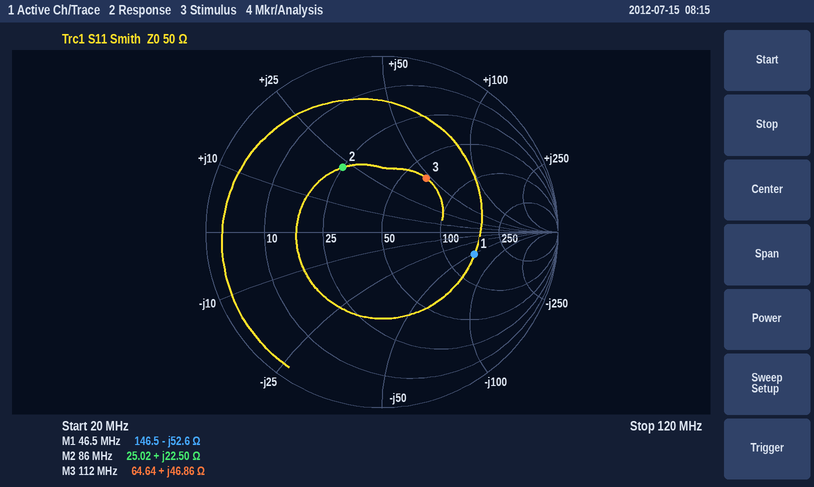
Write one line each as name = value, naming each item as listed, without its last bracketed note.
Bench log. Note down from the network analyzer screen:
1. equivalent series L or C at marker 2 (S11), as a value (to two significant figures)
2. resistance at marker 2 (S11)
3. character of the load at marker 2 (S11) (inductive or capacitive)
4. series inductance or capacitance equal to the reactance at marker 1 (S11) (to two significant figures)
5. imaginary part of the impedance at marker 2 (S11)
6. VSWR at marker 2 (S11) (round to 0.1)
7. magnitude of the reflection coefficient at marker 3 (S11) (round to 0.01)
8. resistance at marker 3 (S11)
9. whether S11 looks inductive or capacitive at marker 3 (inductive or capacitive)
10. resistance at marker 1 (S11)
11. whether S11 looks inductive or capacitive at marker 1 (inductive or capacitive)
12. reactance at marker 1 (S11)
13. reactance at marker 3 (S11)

equivalent series L or C at marker 2 (S11), as a value = 42 nH
resistance at marker 2 = 25.02 Ω
character of the load at marker 2 (S11) = inductive
series inductance or capacitance equal to the reactance at marker 1 (S11) = 65 pF
imaginary part of the impedance at marker 2 = +22.50 Ω
VSWR at marker 2 (S11) = 2.5
magnitude of the reflection coefficient at marker 3 (S11) = 0.40
resistance at marker 3 = 64.64 Ω
whether S11 looks inductive or capacitive at marker 3 = inductive
resistance at marker 1 = 146.5 Ω
whether S11 looks inductive or capacitive at marker 1 = capacitive
reactance at marker 1 = -52.6 Ω
reactance at marker 3 = +46.86 Ω
